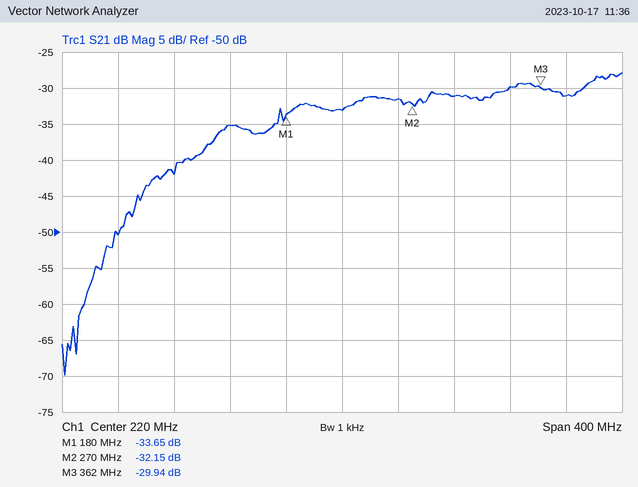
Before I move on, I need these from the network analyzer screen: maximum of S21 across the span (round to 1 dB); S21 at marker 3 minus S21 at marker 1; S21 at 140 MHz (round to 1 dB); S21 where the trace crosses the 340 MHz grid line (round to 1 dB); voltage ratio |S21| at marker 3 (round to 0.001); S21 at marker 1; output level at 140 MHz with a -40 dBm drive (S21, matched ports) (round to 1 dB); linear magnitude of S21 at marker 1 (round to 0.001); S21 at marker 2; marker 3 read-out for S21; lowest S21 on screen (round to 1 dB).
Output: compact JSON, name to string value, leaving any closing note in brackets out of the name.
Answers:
{"maximum of S21 across the span": "-28 dB", "S21 at marker 3 minus S21 at marker 1": "3.71 dB", "S21 at 140 MHz": "-35 dB", "S21 where the trace crosses the 340 MHz grid line": "-30 dB", "voltage ratio |S21| at marker 3": "0.032", "S21 at marker 1": "-33.65 dB", "output level at 140 MHz with a -40 dBm drive (S21, matched ports)": "-75 dBm", "linear magnitude of S21 at marker 1": "0.021", "S21 at marker 2": "-32.15 dB", "marker 3 read-out for S21": "-29.94 dB", "lowest S21 on screen": "-70 dB"}
